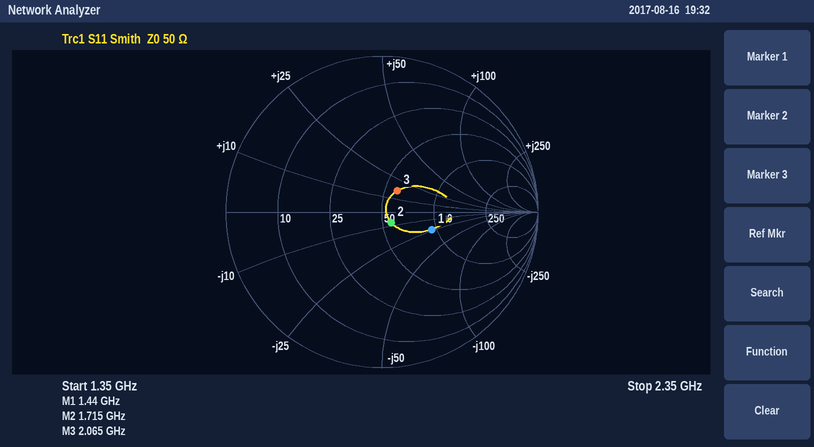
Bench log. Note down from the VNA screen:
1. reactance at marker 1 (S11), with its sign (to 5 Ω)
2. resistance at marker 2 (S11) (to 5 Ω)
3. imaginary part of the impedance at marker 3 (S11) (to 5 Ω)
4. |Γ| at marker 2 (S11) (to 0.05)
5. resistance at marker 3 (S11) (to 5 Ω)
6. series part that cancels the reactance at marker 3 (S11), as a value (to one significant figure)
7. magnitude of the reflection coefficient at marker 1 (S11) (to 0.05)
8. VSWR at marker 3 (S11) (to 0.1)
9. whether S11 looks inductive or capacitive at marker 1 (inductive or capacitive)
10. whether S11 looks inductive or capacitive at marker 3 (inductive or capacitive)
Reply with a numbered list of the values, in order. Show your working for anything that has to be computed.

1. -25 Ω
2. 55 Ω
3. +15 Ω
4. 0.10
5. 60 Ω
6. C = 1/(2π × 2.065 GHz × 15 Ω) ≈ 5 pF
7. 0.35
8. 1.4
9. capacitive
10. inductive
